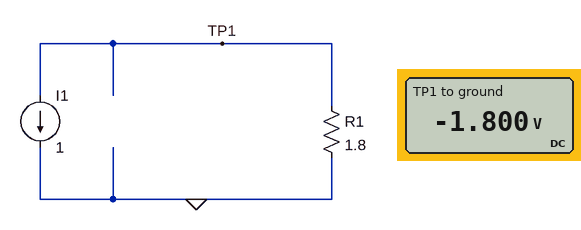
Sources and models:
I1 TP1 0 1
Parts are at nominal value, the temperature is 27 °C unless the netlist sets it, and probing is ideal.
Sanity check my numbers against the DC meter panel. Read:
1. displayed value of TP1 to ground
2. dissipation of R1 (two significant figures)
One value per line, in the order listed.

-1.800 V
1.8 W
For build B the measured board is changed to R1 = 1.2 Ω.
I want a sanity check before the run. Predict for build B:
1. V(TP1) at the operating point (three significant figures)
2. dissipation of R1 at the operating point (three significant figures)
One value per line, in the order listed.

-1.20 V
1.20 W
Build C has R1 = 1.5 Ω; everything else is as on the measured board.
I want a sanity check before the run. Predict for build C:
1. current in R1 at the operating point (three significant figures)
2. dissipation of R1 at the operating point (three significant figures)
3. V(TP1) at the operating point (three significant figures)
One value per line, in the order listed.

1.00 A
1.50 W
-1.50 V
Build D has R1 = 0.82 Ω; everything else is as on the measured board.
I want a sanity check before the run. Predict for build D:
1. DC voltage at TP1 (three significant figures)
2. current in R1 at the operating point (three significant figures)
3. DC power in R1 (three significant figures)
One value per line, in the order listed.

-820 mV
1.00 A
820 mW
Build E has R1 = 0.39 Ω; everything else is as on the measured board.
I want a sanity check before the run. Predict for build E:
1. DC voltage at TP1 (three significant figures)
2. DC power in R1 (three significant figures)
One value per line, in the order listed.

-390 mV
390 mW
